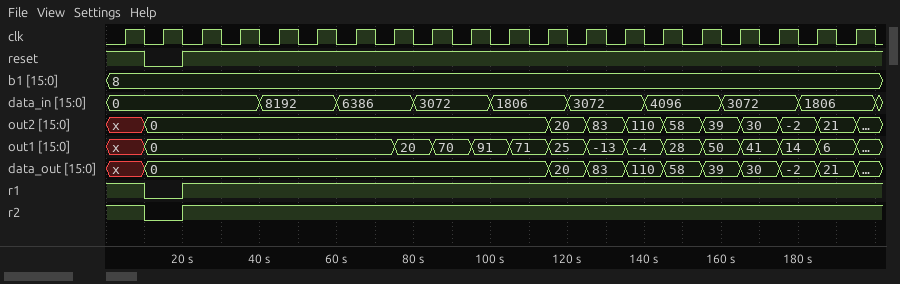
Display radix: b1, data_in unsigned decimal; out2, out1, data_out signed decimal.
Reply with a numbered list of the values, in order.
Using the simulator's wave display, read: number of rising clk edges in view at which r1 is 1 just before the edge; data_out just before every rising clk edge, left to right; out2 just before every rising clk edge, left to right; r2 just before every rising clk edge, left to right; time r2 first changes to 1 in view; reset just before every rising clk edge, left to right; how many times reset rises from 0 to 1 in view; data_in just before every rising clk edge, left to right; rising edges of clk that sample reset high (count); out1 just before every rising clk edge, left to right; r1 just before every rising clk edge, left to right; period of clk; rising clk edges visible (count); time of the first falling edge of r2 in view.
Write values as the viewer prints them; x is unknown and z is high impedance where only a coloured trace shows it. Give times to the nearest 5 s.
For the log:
1. 19
2. x, 0, 0, 0, 0, 0, 0, 0, 0, 0, 0, 0, 20, 83, 110, 58, 39, 30, -2, 21
3. x, 0, 0, 0, 0, 0, 0, 0, 0, 0, 0, 0, 20, 83, 110, 58, 39, 30, -2, 21
4. 1 0 1 1 1 1 1 1 1 1 1 1 1 1 1 1 1 1 1 1
5. 20 s
6. 1 0 1 1 1 1 1 1 1 1 1 1 1 1 1 1 1 1 1 1
7. 1
8. 0, 0, 0, 0, 8192, 8192, 6386, 6386, 3072, 3072, 1806, 1806, 3072, 3072, 4096, 4096, 3072, 3072, 1806, 1806
9. 19
10. x, 0, 0, 0, 0, 0, 0, 0, 20, 70, 91, 71, 25, -13, -4, 28, 50, 41, 14, 6
11. 1 0 1 1 1 1 1 1 1 1 1 1 1 1 1 1 1 1 1 1
12. 10 s
13. 20
14. 10 s
